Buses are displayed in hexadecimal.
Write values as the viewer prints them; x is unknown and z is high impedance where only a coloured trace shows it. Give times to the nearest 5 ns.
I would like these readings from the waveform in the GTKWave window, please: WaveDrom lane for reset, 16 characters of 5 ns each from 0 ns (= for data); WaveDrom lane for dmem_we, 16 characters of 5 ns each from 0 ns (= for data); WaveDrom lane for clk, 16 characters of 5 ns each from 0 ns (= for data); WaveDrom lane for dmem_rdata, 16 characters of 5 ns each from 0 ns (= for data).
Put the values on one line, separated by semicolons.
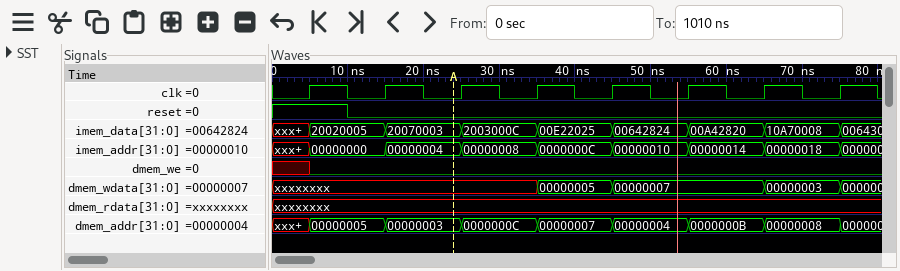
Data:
{name: 'reset', wave: '1.0.............'}; {name: 'dmem_we', wave: 'x0..............'}; {name: 'clk', wave: '0101010101010101'}; {name: 'dmem_rdata', wave: 'x...............'}
